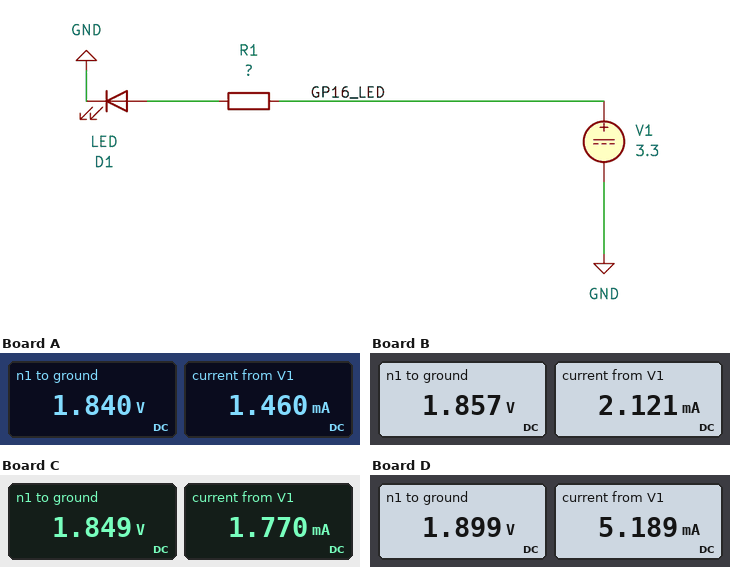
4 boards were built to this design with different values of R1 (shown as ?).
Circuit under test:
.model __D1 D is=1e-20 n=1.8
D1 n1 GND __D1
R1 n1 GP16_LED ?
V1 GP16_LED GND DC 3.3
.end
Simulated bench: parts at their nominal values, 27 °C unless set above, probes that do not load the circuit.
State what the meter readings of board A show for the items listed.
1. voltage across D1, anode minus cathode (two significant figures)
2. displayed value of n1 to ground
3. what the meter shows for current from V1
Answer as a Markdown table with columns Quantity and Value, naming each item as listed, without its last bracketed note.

| Quantity | Value |
|---|---|
| voltage across D1, anode minus cathode | 1.8 V |
| displayed value of n1 to ground | 1.840 V |
| what the meter shows for current from V1 | 1.460 mA |
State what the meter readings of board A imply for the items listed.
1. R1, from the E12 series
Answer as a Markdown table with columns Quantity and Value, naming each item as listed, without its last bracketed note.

| Quantity | Value |
|---|---|
| R1, from the E12 series | 1 kΩ |
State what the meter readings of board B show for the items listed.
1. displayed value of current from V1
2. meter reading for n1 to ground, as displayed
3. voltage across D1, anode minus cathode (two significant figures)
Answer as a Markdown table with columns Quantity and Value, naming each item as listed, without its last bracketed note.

| Quantity | Value |
|---|---|
| displayed value of current from V1 | 2.121 mA |
| meter reading for n1 to ground, as displayed | 1.857 V |
| voltage across D1, anode minus cathode | 1.9 V |
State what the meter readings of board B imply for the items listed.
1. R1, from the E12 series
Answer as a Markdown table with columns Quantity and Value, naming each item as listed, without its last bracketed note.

| Quantity | Value |
|---|---|
| R1, from the E12 series | 680 Ω |
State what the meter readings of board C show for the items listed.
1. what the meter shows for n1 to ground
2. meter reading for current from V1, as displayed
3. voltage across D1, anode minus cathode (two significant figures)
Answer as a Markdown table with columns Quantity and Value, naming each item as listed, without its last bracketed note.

| Quantity | Value |
|---|---|
| what the meter shows for n1 to ground | 1.849 V |
| meter reading for current from V1, as displayed | 1.770 mA |
| voltage across D1, anode minus cathode | 1.8 V |
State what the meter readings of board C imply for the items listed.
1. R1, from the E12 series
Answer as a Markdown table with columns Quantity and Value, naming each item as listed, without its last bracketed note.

| Quantity | Value |
|---|---|
| R1, from the E12 series | 820 Ω |
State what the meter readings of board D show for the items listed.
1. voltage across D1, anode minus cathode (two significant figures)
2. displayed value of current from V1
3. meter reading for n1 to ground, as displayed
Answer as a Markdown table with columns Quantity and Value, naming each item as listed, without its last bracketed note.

| Quantity | Value |
|---|---|
| voltage across D1, anode minus cathode | 1.9 V |
| displayed value of current from V1 | 5.189 mA |
| meter reading for n1 to ground, as displayed | 1.899 V |
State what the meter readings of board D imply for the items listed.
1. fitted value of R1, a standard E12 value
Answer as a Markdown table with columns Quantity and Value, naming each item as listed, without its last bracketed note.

| Quantity | Value |
|---|---|
| fitted value of R1, a standard E12 value | 270 Ω |
